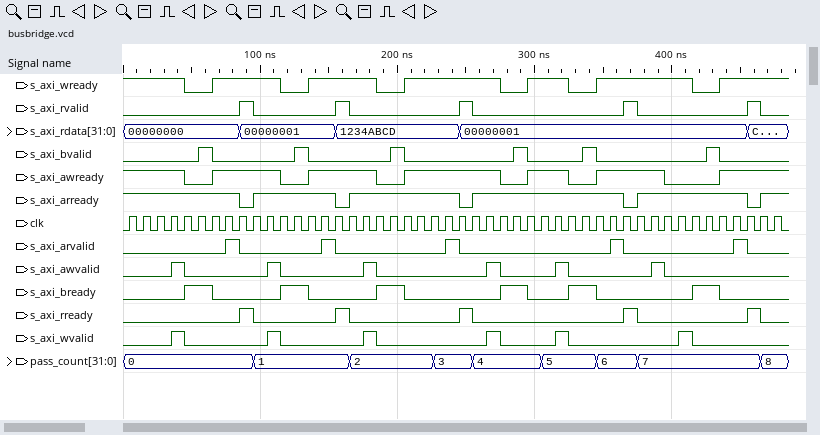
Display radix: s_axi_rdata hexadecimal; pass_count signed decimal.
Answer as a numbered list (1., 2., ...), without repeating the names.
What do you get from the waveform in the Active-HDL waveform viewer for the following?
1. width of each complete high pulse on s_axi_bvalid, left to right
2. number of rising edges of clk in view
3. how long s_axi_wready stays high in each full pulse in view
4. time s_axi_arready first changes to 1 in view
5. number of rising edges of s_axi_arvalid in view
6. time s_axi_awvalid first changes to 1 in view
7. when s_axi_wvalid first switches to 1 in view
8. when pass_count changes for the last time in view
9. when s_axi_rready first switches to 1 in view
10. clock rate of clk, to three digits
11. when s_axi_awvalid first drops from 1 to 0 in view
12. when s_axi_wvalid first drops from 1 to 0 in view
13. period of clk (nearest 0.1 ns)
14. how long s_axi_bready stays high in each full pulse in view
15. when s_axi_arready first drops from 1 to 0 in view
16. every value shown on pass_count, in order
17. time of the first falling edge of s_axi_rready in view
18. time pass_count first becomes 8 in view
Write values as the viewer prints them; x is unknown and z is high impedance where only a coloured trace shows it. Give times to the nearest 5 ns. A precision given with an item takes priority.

1. 10 ns, 10 ns, 10 ns, 10 ns, 10 ns, 10 ns
2. 48
3. 50 ns, 50 ns, 70 ns, 30 ns, 70 ns
4. 95 ns
5. 5
6. 35 ns
7. 35 ns
8. 465 ns
9. 85 ns
10. 100 MHz
11. 45 ns
12. 45 ns
13. 10 ns
14. 20 ns, 20 ns, 20 ns, 20 ns, 20 ns, 20 ns
15. 85 ns
16. 0, 1, 2, 3, 4, 5, 6, 7, 8
17. 95 ns
18. 465 ns
